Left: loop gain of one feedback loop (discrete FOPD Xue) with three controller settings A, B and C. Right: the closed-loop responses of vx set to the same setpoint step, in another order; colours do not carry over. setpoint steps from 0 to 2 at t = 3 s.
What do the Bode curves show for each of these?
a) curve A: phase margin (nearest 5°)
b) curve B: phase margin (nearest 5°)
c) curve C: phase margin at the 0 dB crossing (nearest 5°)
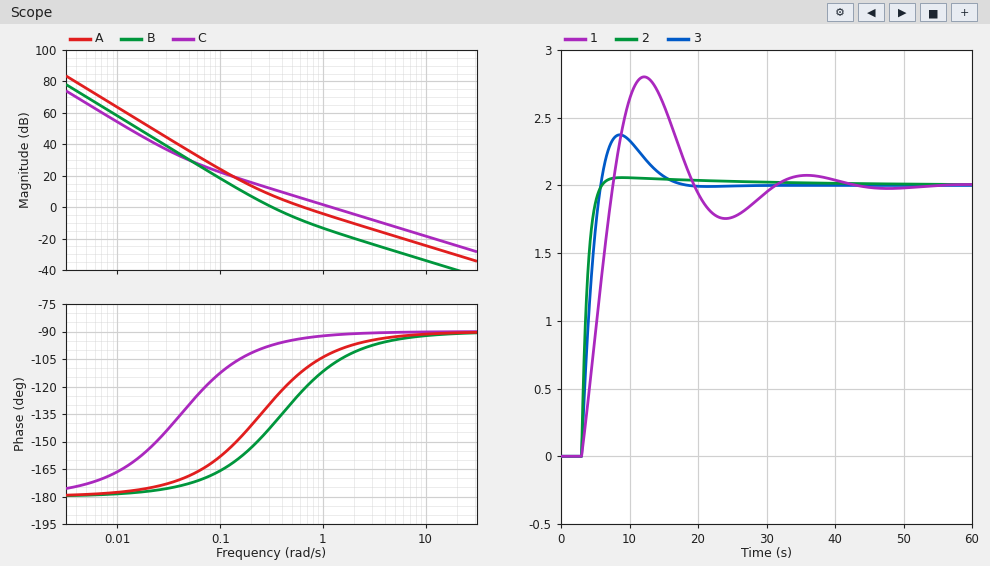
70°
40°
90°
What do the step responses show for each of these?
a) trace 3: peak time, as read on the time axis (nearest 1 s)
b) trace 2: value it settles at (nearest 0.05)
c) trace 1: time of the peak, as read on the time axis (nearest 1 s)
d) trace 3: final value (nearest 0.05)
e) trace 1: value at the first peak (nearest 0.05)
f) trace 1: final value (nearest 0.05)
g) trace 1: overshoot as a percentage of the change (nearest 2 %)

9 s
2.00
12 s
2.00
2.80
2.00
40 %
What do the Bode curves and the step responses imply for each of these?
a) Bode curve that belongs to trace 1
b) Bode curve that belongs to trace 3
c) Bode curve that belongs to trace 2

B
A
C
